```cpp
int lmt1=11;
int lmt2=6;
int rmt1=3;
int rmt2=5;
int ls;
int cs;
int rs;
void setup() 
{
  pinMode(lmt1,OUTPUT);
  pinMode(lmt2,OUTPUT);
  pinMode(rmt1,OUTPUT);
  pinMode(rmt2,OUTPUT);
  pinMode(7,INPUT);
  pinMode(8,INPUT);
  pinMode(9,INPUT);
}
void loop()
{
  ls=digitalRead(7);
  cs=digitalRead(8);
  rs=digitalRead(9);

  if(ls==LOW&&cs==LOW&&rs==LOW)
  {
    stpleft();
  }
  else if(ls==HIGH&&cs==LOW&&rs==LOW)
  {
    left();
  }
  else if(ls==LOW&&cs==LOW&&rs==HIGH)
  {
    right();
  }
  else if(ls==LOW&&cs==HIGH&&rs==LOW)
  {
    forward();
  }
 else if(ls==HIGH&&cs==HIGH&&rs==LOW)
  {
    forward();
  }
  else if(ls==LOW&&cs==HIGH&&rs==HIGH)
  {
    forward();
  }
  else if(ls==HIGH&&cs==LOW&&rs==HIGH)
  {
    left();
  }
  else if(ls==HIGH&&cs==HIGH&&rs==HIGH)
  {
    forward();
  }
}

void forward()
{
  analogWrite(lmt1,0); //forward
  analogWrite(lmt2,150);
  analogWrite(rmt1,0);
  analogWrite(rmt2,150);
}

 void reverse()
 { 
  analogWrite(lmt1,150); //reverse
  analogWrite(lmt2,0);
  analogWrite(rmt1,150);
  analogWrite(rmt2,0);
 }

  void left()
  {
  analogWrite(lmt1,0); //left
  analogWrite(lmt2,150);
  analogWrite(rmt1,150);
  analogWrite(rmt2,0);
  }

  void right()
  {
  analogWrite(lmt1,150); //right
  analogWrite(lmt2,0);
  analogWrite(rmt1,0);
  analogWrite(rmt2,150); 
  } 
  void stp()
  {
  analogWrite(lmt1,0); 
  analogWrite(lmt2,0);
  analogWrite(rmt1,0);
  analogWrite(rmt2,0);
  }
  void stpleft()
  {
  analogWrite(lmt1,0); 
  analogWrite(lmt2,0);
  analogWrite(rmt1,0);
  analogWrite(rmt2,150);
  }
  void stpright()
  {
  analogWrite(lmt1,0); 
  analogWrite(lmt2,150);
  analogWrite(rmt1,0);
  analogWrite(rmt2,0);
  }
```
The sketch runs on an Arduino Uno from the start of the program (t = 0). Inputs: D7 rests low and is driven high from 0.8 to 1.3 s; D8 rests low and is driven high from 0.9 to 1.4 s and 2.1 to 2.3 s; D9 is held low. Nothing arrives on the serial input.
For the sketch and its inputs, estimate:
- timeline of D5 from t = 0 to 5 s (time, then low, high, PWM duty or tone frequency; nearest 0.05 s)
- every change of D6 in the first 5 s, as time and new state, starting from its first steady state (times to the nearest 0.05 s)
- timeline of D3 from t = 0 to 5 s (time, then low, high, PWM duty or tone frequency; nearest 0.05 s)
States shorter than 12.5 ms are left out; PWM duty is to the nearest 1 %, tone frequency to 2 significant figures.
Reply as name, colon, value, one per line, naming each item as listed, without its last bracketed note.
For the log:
timeline of D5 from t = 0 to 5 s: 0 s PWM 59 %; 0.8 s low; 0.9 s PWM 59 %
every change of D6 in the first 5 s, as time and new state, starting from its first steady state: 0 s low; 0.8 s PWM 59 %; 1.4 s low; 2.1 s PWM 59 %; 2.3 s low
timeline of D3 from t = 0 to 5 s: 0 s low; 0.8 s PWM 59 %; 0.9 s low
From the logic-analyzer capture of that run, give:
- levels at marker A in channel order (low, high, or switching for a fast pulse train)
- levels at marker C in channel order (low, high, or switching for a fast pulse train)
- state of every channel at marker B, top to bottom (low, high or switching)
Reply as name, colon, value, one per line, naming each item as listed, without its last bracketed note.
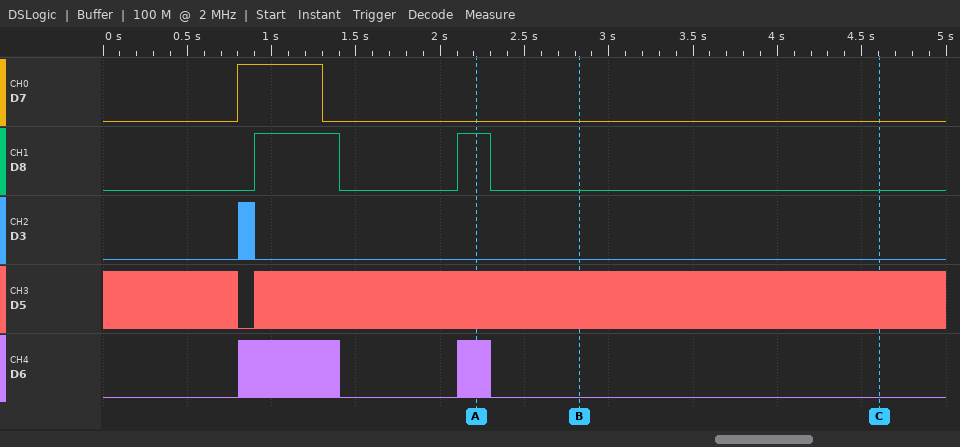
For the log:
levels at marker A in channel order: D7 low, D8 high, D3 low, D5 switching, D6 switching
levels at marker C in channel order: D7 low, D8 low, D3 low, D5 switching, D6 low
state of every channel at marker B, top to bottom: D7 low, D8 low, D3 low, D5 switching, D6 low
